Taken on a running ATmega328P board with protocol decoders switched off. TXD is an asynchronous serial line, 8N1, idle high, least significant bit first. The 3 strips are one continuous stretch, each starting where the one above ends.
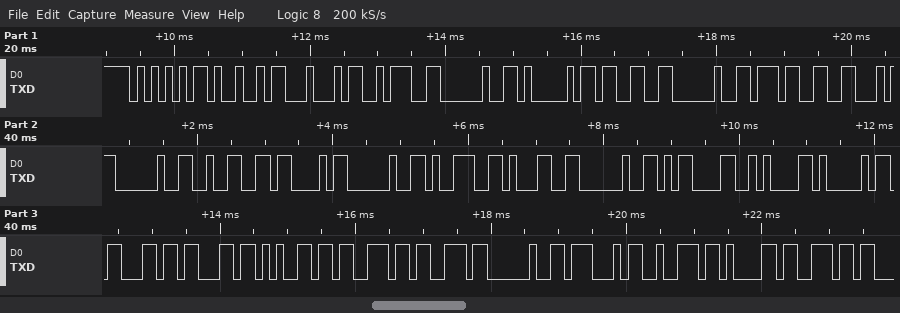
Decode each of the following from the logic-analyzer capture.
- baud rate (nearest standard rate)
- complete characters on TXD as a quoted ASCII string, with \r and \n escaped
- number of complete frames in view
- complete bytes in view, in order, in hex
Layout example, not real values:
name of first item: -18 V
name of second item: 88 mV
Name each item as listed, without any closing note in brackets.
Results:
baud rate: 9600 baud
complete characters on TXD as a quoted ASCII string, with \r and \n escaped: "UID: A3 7F 2C 91 \r\nAccess Gran"
number of complete frames in view: 30
complete bytes in view, in order, in hex: 55 49 44 3A 20 41 33 20 37 46 20 32 43 20 39 31 20 0D 0A 41 63 63 65 73 73 20 47 72 61 6E
